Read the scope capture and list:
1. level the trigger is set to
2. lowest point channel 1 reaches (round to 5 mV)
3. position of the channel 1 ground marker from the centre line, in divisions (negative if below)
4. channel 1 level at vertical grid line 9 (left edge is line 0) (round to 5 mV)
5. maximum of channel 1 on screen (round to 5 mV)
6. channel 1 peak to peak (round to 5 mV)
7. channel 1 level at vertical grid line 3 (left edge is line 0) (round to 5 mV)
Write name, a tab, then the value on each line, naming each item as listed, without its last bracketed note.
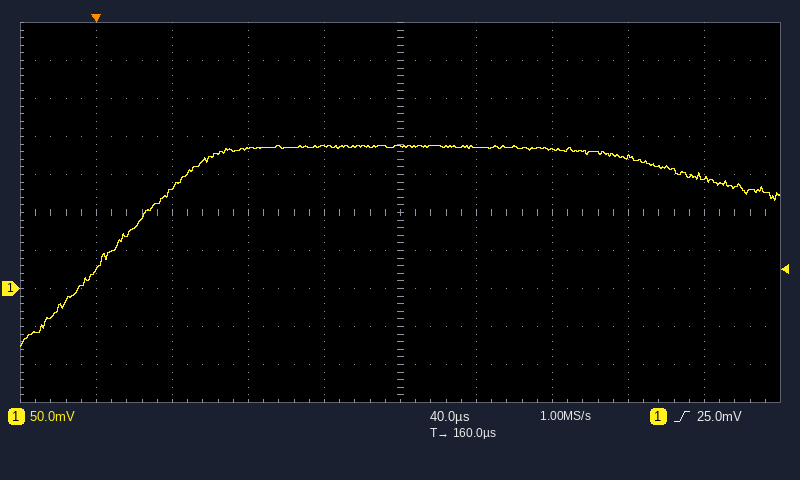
level the trigger is set to	25.0 mV
lowest point channel 1 reaches	-75 mV
position of the channel 1 ground marker from the centre line, in divisions	-2.0 div
channel 1 level at vertical grid line 9 (left edge is line 0)	145 mV
maximum of channel 1 on screen	190 mV
channel 1 peak to peak	265 mV
channel 1 level at vertical grid line 3 (left edge is line 0)	185 mV
